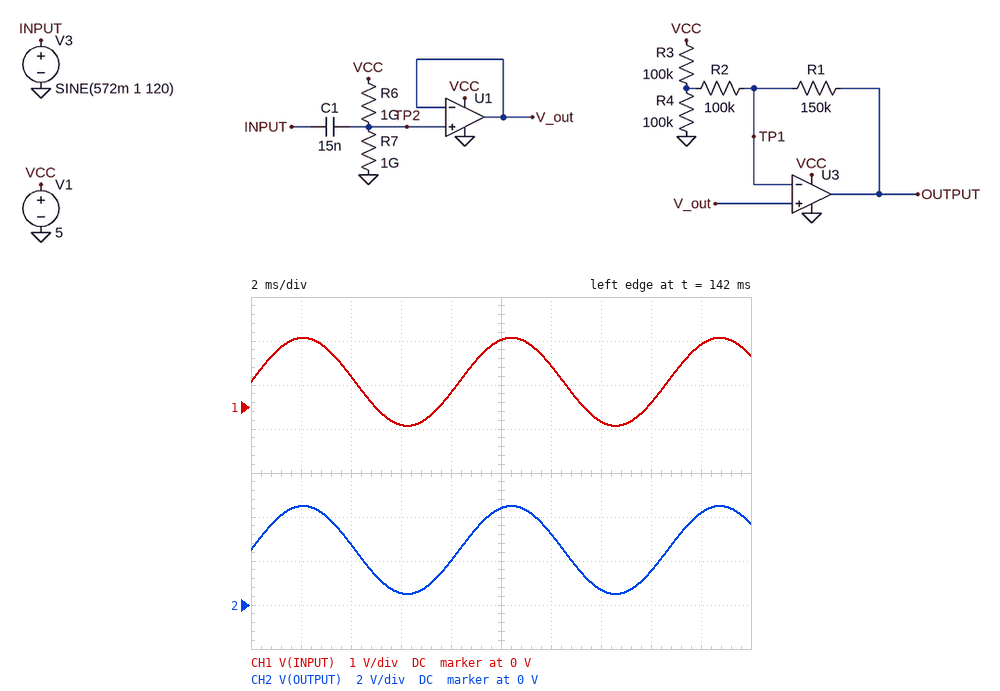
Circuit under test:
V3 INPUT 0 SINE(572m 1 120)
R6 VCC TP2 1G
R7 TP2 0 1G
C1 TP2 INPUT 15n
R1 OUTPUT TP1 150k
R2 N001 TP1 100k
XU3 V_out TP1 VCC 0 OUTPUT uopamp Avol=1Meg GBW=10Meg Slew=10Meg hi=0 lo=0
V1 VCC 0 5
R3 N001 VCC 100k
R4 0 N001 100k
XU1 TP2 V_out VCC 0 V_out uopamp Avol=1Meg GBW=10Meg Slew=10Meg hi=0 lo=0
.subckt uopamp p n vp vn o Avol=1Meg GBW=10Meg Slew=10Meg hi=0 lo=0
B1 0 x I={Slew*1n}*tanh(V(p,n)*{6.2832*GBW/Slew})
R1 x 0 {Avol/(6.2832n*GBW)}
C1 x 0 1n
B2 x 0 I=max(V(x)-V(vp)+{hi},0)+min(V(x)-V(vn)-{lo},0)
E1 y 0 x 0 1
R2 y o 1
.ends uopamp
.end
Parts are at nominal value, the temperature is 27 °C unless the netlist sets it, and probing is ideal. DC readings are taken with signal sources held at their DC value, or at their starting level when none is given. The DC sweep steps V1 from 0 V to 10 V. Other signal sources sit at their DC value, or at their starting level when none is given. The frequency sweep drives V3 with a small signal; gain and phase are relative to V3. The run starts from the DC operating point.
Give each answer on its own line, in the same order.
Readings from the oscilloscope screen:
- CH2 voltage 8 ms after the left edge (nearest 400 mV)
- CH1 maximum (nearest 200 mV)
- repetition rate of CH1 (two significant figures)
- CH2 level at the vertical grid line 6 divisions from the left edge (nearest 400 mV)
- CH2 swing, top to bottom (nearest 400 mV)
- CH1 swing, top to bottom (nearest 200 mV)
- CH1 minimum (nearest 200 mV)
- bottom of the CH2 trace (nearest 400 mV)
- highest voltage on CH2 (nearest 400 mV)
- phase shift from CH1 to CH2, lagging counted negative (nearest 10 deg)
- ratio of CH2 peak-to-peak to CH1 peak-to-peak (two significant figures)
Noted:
2.0 V
1.6 V
120 Hz
3.2 V
4.0 V
2.0 V
-400 mV
400 mV
4.4 V
0 deg
2.0
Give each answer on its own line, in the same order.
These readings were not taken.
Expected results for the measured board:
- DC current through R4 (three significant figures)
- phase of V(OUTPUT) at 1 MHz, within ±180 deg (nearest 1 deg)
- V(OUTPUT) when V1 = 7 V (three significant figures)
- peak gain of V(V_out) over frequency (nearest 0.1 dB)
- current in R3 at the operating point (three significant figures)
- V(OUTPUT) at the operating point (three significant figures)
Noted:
25.0 µA
-17 deg
3.50 V
0 dB
25.0 µA
2.50 V
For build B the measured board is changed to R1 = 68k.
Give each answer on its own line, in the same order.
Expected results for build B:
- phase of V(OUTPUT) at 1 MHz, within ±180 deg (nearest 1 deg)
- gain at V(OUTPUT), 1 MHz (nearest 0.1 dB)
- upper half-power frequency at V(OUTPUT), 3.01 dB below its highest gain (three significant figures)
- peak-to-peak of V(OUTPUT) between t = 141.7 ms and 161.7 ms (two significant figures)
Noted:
-14 deg
3.1 dB
5.21 MHz
2.9 V
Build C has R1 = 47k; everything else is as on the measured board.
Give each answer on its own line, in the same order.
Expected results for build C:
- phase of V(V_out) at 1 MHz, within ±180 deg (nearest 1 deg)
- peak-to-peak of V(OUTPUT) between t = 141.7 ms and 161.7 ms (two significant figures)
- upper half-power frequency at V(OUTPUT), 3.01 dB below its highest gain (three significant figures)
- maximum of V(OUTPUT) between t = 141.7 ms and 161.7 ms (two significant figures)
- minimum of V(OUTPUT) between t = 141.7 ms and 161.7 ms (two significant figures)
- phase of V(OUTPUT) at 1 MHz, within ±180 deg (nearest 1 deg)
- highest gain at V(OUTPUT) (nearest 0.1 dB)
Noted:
-6 deg
2.6 V
5.54 MHz
3.8 V
1.2 V
-13 deg
2.4 dB
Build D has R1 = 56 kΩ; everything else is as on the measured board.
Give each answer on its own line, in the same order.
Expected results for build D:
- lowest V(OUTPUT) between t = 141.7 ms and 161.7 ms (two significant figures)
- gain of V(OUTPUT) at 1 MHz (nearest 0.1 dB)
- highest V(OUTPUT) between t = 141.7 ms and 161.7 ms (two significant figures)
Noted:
1.1 V
2.6 dB
3.9 V
